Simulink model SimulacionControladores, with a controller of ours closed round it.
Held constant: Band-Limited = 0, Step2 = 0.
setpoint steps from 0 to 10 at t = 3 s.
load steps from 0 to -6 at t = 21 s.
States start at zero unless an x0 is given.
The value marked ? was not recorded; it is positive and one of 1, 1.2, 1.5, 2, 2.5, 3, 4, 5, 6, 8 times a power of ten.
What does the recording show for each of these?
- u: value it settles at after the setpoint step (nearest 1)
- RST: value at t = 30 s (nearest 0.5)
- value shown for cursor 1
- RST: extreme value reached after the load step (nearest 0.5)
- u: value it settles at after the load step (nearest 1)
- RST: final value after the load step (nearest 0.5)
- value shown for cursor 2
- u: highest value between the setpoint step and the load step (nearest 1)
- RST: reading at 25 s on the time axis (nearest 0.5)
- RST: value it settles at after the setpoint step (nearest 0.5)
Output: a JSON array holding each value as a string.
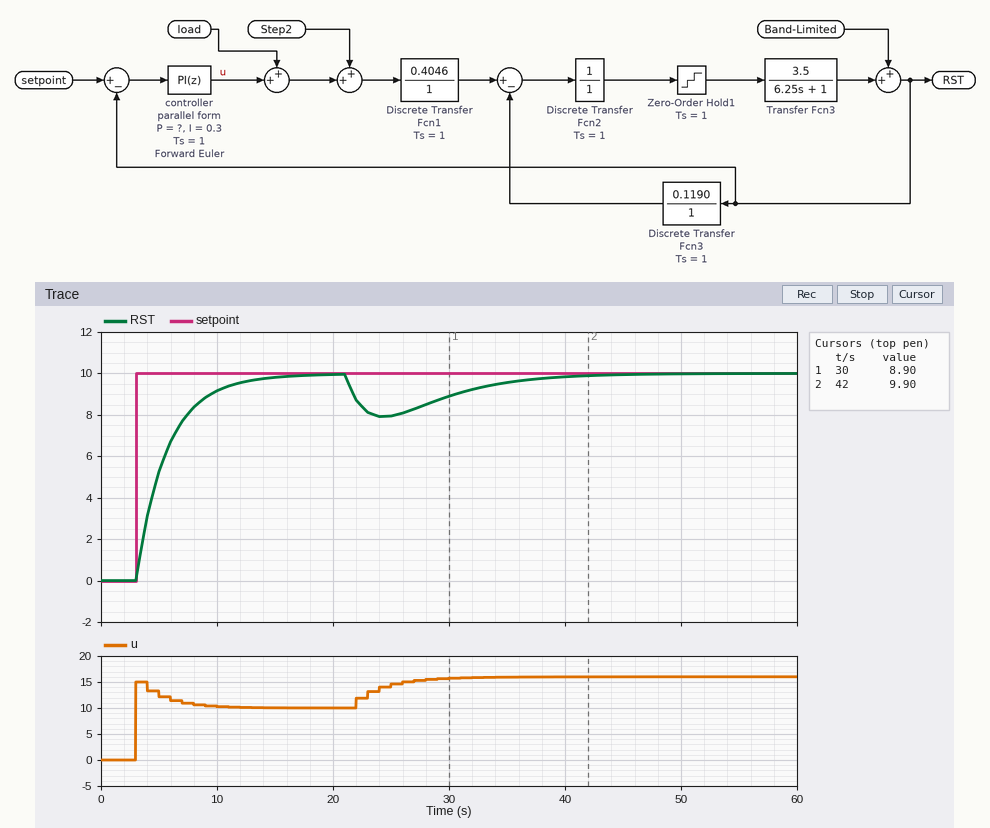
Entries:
["10", "9.0", "8.90", "8.0", "16", "10.0", "9.90", "15", "8.0", "10.0"]
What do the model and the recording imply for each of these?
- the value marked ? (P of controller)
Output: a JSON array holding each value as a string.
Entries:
["1.5"]
